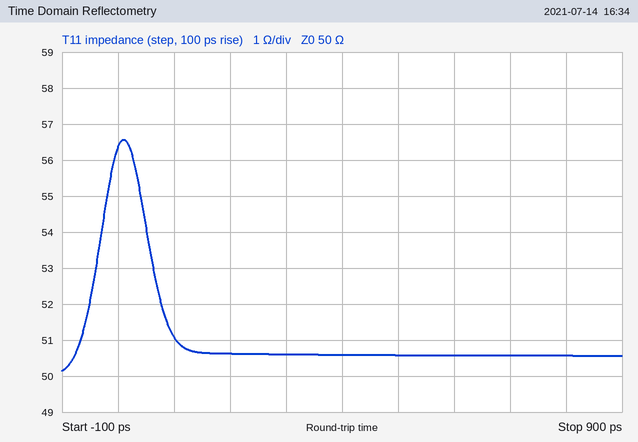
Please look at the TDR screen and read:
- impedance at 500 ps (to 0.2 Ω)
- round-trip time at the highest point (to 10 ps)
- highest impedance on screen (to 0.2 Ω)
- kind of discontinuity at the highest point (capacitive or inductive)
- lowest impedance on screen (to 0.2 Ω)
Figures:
50.6 Ω
10 ps
56.6 Ω
inductive
50.2 Ω
